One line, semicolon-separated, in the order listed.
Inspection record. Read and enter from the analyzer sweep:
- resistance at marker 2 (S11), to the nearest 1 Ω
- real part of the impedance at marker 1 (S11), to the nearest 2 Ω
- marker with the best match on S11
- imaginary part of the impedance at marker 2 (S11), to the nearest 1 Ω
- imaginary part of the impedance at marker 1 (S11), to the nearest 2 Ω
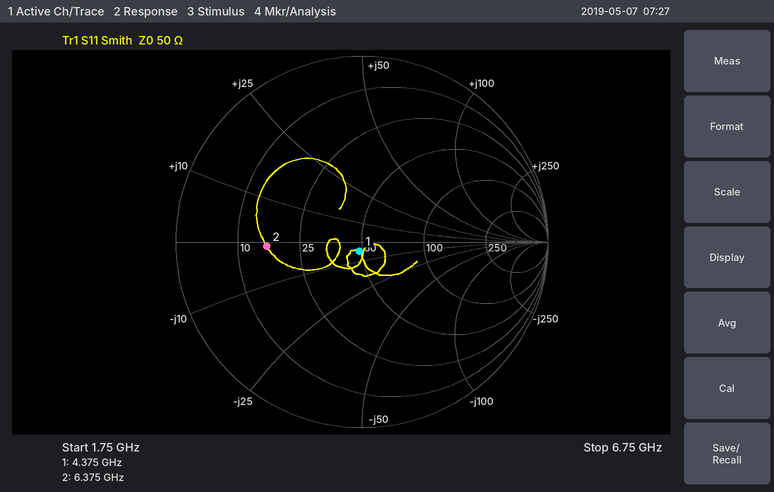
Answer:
16 Ω; 48 Ω; marker 1; -1 Ω; -4 Ω
